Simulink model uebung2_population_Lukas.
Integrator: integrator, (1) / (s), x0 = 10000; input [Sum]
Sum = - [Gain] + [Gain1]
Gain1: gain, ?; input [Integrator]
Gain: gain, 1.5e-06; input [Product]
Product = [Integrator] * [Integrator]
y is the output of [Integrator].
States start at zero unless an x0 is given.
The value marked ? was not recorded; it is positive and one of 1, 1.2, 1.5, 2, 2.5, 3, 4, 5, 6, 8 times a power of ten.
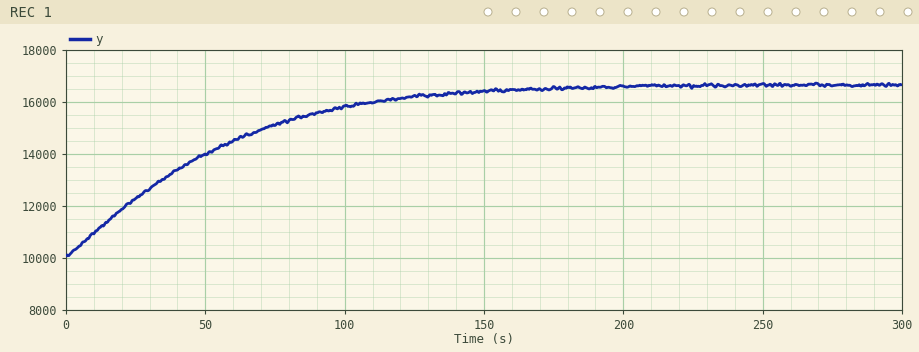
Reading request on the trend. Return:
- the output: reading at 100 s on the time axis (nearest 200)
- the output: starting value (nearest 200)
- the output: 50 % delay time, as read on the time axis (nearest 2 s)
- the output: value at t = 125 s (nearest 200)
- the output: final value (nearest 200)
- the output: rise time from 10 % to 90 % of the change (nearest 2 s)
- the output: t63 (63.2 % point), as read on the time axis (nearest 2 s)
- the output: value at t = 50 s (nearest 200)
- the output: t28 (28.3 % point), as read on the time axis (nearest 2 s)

15800
10000
40 s
16200
16600
104 s
54 s
14000
20 s
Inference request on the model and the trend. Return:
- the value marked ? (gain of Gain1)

0.025
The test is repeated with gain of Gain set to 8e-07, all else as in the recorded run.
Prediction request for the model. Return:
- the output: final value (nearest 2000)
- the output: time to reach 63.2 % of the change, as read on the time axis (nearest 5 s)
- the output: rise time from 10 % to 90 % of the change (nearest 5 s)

32000
75 s
125 s
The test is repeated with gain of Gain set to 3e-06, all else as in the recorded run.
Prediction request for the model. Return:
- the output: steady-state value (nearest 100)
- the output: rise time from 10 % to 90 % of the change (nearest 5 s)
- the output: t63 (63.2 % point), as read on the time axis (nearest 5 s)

8300
80 s
35 s
